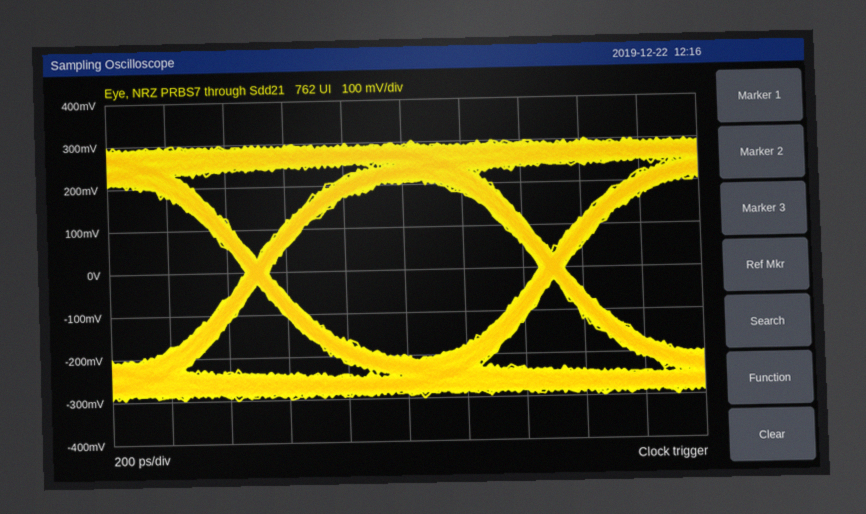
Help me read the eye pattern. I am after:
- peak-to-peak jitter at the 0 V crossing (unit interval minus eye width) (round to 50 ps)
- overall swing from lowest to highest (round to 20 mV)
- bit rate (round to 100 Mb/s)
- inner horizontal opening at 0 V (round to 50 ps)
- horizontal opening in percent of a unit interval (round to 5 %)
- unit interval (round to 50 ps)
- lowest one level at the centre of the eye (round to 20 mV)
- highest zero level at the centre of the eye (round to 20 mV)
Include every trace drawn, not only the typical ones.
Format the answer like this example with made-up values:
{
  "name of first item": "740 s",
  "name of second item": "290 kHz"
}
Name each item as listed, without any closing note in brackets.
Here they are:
{
  "peak-to-peak jitter at the 0 V crossing (unit interval minus eye width)": "100 ps",
  "overall swing from lowest to highest": "600 mV",
  "bit rate": "1.0 Gb/s",
  "inner horizontal opening at 0 V": "900 ps",
  "horizontal opening in percent of a unit interval": "90 %",
  "unit interval": "1.00 ns",
  "lowest one level at the centre of the eye": "200 mV",
  "highest zero level at the centre of the eye": "-200 mV"
}
